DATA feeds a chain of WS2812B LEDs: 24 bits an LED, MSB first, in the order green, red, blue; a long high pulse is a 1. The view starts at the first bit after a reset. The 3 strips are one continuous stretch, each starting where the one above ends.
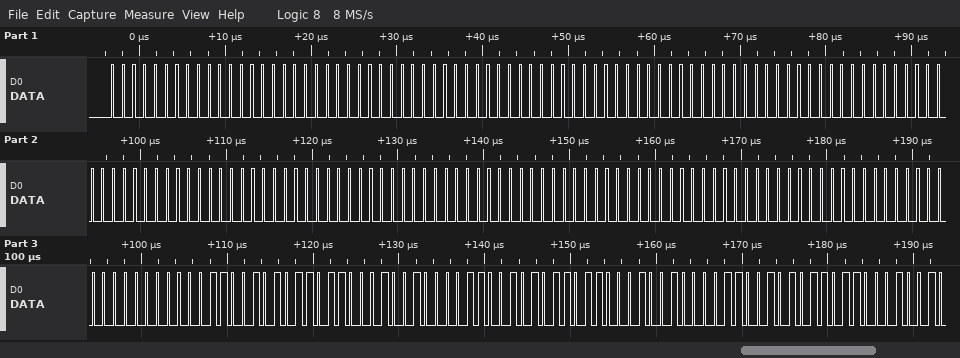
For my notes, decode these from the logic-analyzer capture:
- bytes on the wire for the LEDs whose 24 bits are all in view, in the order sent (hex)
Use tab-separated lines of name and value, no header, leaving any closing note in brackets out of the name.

bytes on the wire for the LEDs whose 24 bits are all in view, in the order sent	00 00 00 00 00 00 00 00 00 00 00 00 00 00 00 00 00 00 00 00 00 65 6C 48 65 6C 48
